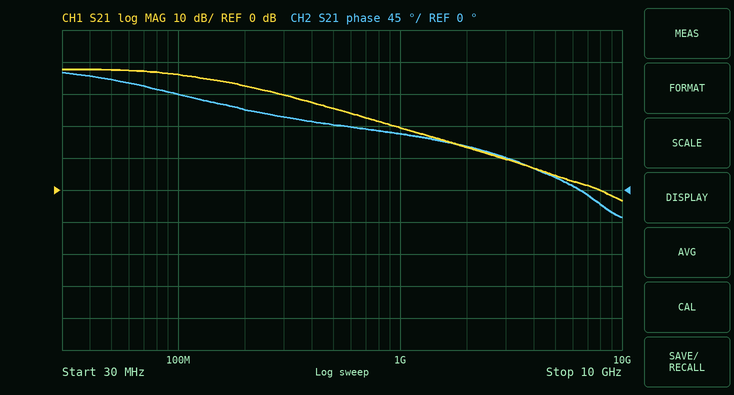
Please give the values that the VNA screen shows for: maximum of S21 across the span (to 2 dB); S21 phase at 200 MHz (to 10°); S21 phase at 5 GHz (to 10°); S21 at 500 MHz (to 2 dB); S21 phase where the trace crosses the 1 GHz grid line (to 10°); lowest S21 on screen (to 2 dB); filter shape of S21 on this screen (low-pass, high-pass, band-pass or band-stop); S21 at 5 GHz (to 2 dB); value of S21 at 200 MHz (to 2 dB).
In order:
38 dB
110°
20°
26 dB
80°
-4 dB
low-pass
4 dB
32 dB
